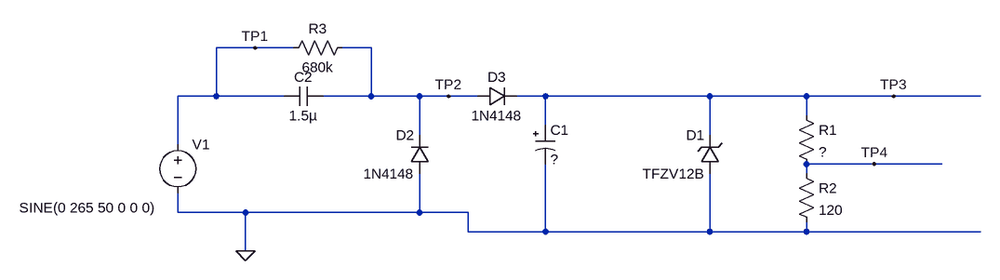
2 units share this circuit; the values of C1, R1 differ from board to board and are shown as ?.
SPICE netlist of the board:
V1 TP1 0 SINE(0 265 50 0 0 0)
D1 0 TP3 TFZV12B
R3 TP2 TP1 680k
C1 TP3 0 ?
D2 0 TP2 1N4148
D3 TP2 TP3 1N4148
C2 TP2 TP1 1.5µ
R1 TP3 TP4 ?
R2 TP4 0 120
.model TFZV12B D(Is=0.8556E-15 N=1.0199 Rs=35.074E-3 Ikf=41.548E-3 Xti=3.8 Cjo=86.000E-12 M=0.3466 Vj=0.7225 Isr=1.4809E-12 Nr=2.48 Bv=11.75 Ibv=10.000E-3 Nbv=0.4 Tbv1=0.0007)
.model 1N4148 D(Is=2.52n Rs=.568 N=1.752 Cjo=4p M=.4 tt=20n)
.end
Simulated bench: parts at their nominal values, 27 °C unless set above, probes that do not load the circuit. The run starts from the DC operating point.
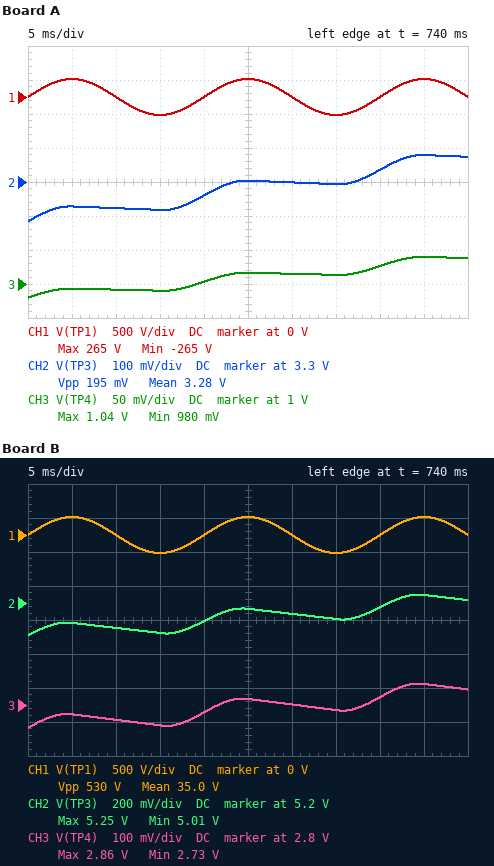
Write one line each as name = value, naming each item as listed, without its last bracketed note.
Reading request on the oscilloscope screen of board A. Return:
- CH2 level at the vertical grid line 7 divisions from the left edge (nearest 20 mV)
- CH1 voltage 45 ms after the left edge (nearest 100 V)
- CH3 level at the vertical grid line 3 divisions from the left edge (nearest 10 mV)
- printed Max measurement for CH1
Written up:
CH2 level at the vertical grid line 7 divisions from the left edge = 3.30 V
CH1 voltage 45 ms after the left edge = 300 V
CH3 level at the vertical grid line 3 divisions from the left edge = 990 mV
printed Max measurement for CH1 = 265 V
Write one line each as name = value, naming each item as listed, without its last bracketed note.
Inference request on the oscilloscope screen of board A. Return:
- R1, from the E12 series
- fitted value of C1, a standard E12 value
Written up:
R1, from the E12 series = 270 Ω
fitted value of C1, a standard E12 value = 8.2 mF
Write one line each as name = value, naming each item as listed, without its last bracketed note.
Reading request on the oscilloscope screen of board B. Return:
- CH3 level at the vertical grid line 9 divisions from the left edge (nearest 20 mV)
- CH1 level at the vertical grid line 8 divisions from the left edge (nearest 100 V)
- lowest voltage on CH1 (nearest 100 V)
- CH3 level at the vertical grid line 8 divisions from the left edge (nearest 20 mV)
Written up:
CH3 level at the vertical grid line 9 divisions from the left edge = 2.86 V
CH1 level at the vertical grid line 8 divisions from the left edge = 0 V
lowest voltage on CH1 = -300 V
CH3 level at the vertical grid line 8 divisions from the left edge = 2.82 V
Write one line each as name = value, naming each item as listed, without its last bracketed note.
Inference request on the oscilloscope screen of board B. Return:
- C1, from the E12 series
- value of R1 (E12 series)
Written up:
C1, from the E12 series = 3.9 mF
value of R1 = 100 Ω
